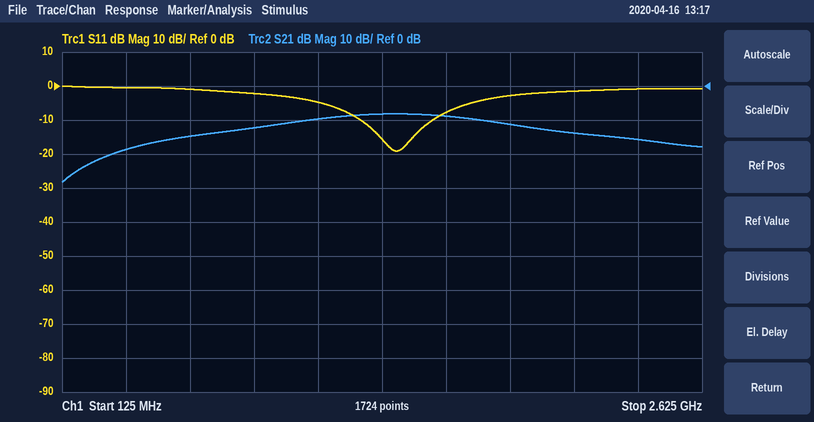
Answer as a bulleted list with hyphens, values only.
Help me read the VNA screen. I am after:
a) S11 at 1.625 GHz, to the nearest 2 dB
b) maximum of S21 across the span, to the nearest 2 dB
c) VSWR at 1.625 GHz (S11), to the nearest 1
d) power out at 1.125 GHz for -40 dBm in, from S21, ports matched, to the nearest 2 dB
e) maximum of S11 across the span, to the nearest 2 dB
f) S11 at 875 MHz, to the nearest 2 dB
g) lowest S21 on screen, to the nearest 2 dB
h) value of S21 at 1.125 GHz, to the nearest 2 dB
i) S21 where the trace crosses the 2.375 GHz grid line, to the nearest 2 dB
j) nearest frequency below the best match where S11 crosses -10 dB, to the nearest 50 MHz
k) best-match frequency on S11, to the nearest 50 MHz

- -8 dB
- -8 dB
- 2
- -50 dBm
- 0 dB
- -2 dB
- -28 dB
- -10 dB
- -16 dB
- 1.30 GHz
- 1.45 GHz
